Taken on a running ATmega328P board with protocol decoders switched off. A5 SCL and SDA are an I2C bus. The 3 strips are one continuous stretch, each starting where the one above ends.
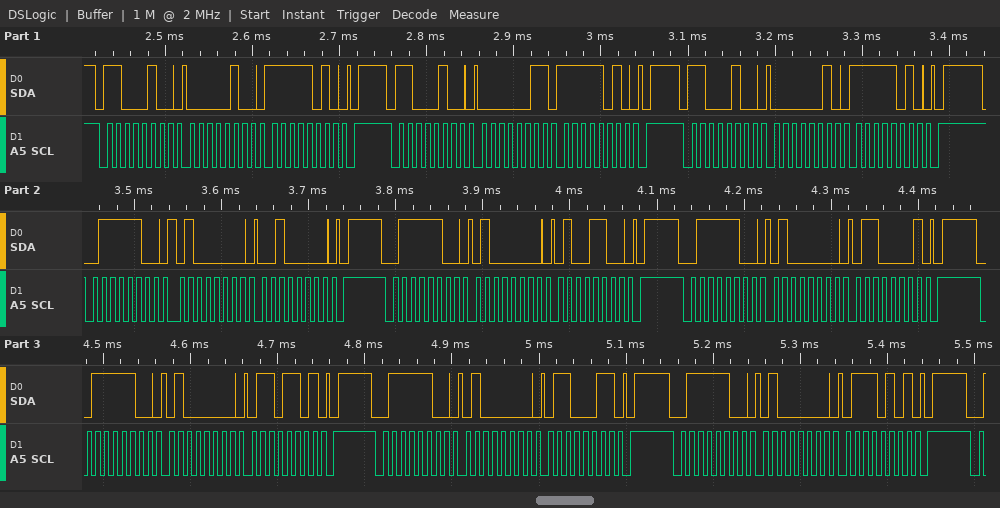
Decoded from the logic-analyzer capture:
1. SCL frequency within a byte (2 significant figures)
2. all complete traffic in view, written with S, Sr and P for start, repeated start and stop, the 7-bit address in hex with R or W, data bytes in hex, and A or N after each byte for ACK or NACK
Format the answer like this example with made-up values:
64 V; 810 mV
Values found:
100 kHz; S 62W A 04 A FA A P S 62W A 03 A FA A P S 62W A 02 A FA A P S 3EW A 40 A 20 A P S 3EW A 40 A 4C A P S 3EW A 40 A 61 A P S 3EW A 40 A 6D A P S 3EW A 40 A 63 A P S 3EW A 40 A 75 A P
